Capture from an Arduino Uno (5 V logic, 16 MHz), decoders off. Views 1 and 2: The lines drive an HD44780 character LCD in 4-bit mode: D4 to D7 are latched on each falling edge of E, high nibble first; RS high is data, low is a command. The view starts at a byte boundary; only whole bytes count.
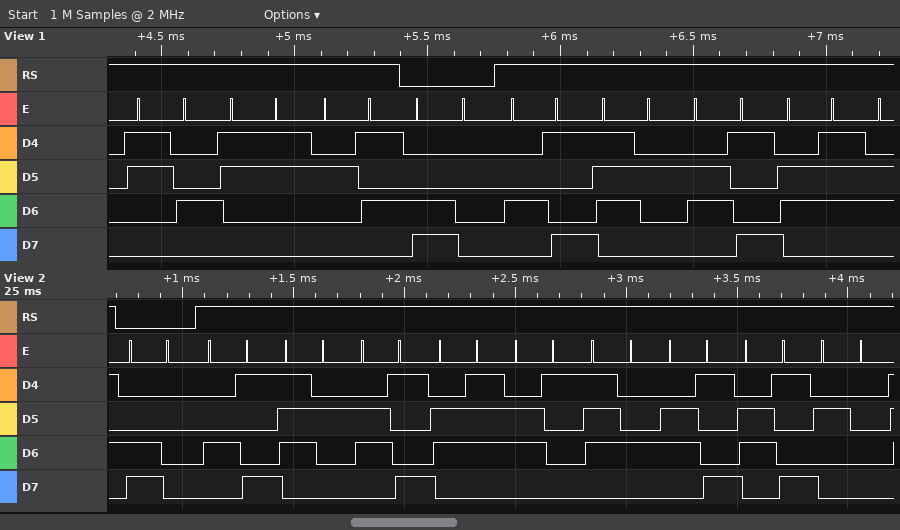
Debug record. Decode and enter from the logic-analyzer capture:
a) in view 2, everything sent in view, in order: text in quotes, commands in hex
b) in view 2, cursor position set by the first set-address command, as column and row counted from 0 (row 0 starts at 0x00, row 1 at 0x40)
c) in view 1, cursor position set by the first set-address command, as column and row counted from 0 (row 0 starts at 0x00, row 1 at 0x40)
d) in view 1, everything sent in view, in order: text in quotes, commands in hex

0xC0 "Irigatii "
column 0, row 1
column 0, row 1
"43%" 0xC0 "Irig"
